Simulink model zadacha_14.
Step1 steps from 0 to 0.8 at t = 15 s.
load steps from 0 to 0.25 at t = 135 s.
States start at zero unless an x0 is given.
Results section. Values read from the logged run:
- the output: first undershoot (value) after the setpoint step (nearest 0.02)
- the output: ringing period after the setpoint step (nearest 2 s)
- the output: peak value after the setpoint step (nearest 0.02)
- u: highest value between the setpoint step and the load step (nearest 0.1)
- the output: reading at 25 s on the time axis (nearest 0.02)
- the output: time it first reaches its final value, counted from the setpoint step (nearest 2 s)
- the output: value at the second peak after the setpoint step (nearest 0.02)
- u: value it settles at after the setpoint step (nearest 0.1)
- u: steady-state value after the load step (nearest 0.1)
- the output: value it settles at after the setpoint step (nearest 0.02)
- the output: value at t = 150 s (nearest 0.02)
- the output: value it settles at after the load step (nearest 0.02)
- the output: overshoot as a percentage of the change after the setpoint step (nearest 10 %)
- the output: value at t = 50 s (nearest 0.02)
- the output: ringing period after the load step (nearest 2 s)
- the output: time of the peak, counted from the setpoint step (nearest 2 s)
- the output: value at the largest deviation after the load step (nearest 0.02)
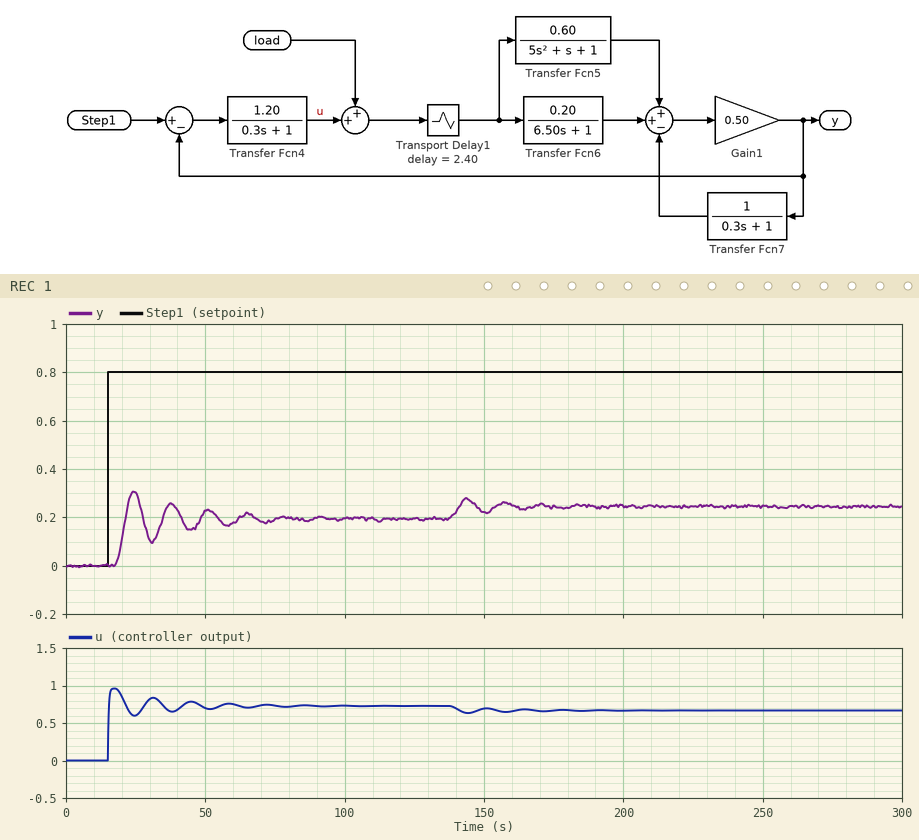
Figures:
0.10
14 s
0.30
1.0
0.30
6 s
0.26
0.7
0.7
0.20
0.22
0.24
60 %
0.22
14 s
10 s
0.28
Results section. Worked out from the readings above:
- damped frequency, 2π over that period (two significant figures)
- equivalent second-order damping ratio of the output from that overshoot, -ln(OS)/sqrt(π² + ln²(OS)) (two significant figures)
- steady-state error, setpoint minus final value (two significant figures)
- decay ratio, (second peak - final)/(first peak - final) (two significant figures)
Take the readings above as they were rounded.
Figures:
0.45 rad/s
0.16
0.60
0.60
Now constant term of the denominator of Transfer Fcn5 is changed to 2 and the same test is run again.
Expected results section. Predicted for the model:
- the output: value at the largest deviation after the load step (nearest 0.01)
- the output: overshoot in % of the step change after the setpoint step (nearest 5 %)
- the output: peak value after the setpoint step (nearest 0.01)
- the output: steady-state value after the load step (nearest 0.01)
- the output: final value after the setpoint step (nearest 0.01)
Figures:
0.18
40 %
0.18
0.17
0.13
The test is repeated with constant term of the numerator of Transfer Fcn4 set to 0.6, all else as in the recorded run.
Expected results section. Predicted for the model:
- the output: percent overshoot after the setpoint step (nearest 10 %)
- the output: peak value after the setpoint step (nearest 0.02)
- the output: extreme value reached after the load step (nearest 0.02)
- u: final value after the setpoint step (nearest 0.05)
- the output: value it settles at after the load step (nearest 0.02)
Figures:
40 %
0.16
0.20
0.40
0.16
